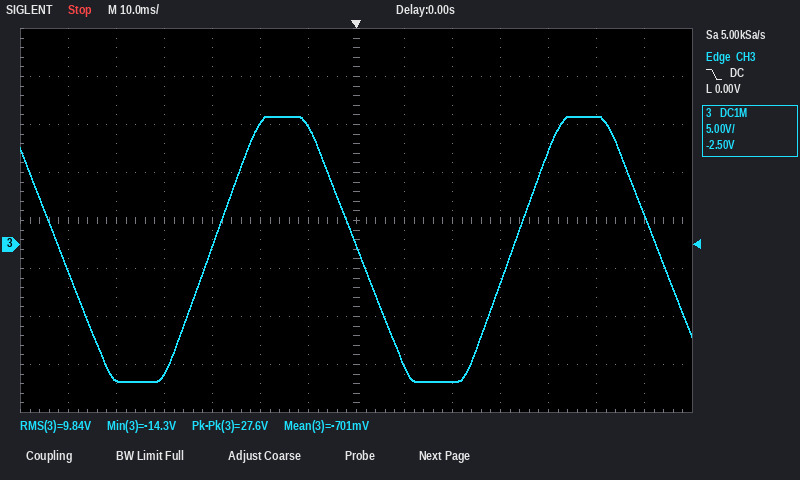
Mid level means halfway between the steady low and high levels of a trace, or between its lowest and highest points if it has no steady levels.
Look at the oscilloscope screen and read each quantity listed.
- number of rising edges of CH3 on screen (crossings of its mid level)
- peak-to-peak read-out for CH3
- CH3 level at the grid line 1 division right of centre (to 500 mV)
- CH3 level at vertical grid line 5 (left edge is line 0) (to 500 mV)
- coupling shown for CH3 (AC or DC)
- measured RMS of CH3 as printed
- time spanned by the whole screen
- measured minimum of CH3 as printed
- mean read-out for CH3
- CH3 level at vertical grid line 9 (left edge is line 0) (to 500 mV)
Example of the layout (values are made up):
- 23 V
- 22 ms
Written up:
- 2
- 27.6 V
- -12.5 V
- 12.5 V
- DC
- 9.84 V
- 140 ms
- -14.3 V
- -701 mV
- -14.5 V
